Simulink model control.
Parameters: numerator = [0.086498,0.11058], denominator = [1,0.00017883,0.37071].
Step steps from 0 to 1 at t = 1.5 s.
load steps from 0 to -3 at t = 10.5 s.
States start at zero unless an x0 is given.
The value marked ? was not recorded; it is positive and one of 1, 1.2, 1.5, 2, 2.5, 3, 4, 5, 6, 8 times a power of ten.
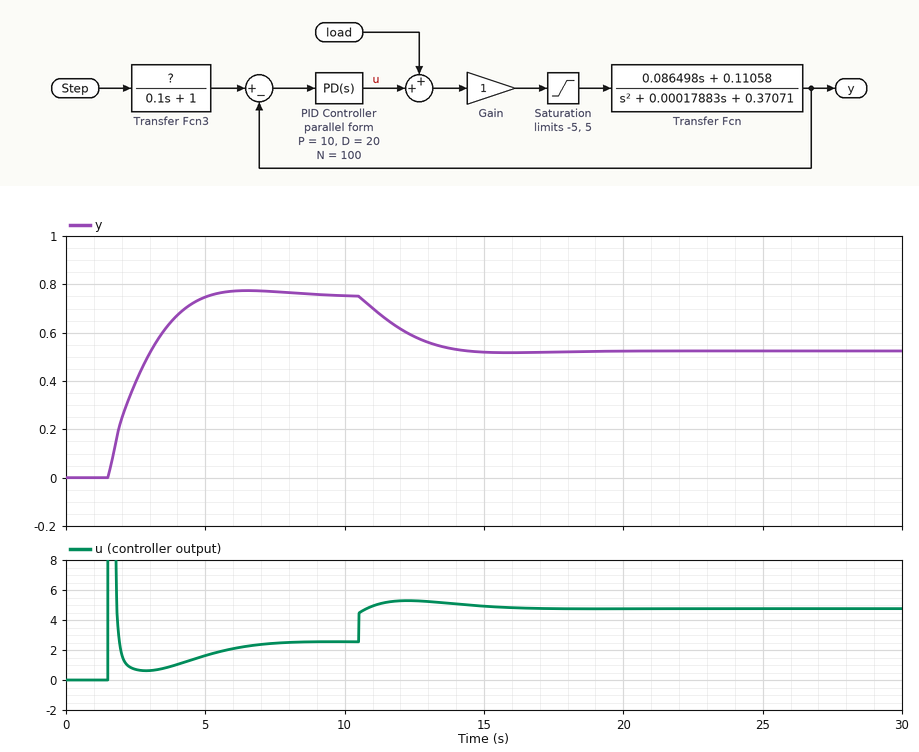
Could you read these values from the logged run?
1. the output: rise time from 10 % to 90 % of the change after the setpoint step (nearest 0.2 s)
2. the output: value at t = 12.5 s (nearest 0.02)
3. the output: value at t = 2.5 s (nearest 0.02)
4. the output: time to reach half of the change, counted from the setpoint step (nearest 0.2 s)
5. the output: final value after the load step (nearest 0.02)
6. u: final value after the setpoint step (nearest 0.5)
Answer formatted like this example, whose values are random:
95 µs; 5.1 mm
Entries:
2.4 s; 0.58; 0.40; 1.0 s; 0.52; 2.5
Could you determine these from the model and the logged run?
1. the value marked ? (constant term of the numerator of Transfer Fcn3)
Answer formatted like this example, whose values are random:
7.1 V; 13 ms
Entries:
1
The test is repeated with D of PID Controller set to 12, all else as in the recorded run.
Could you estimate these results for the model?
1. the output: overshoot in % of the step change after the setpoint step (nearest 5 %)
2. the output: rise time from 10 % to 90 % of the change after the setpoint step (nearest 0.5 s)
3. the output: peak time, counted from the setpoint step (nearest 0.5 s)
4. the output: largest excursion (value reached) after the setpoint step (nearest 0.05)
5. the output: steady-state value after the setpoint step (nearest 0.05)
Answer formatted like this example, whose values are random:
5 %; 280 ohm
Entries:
10 %; 1.5 s; 3.5 s; 0.85; 0.75
